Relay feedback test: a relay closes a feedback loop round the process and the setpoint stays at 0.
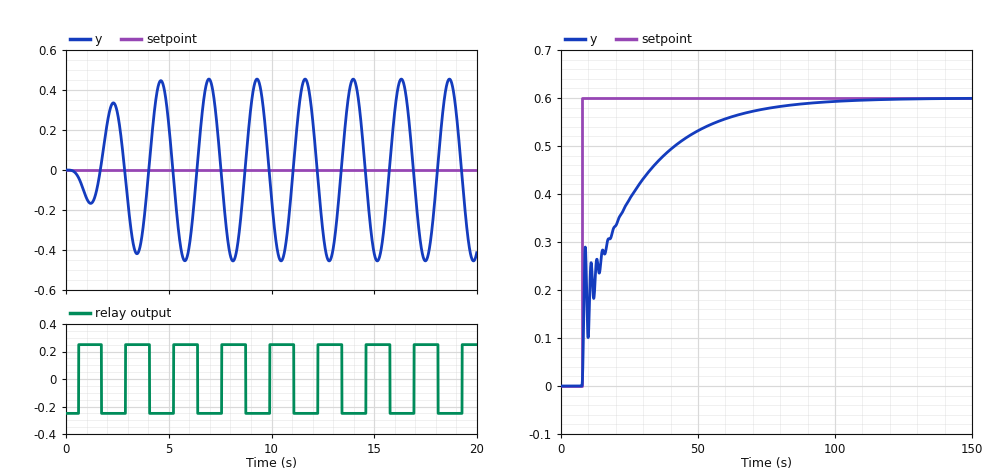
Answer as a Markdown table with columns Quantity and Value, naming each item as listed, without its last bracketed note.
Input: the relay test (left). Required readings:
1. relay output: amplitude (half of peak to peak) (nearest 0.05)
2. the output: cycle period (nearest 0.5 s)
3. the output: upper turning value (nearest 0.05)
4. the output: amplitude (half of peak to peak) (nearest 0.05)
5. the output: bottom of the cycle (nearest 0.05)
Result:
| Quantity | Value |
|---|---|
| relay output: amplitude (half of peak to peak) | 0.25 |
| the output: cycle period | 2.5 s |
| the output: upper turning value | 0.45 |
| the output: amplitude (half of peak to peak) | 0.45 |
| the output: bottom of the cycle | -0.45 |
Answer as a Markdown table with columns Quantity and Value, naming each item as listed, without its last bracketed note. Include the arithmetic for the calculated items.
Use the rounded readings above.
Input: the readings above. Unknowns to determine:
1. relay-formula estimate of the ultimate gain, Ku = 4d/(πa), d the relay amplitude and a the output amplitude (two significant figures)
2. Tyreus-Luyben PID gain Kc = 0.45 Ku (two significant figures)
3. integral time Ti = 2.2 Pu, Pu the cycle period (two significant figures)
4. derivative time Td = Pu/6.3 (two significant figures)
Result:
| Quantity | Value |
|---|---|
| relay-formula estimate of the ultimate gain, Ku = 4d/(πa), d the relay amplitude and a the output amplitude | 4 × 0.25 / (π × 0.45) = 0.71 |
| Tyreus-Luyben PID gain Kc = 0.45 Ku | 0.45 × 0.71 = 0.32 |
| integral time Ti = 2.2 Pu, Pu the cycle period | 2.2 × 2.5 = 5.5 s |
| derivative time Td = Pu/6.3 | 2.5 / 6.3 = 0.40 s |
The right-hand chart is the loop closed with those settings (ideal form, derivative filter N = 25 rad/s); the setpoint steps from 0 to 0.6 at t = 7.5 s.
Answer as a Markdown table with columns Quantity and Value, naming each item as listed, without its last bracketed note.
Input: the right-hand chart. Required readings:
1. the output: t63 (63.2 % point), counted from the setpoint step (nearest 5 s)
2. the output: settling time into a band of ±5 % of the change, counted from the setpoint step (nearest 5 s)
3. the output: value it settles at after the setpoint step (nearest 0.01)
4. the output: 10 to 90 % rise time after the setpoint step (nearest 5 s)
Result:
| Quantity | Value |
|---|---|
| the output: t63 (63.2 % point), counted from the setpoint step | 15 s |
| the output: settling time into a band of ±5 % of the change, counted from the setpoint step | 60 s |
| the output: value it settles at after the setpoint step | 0.60 |
| the output: 10 to 90 % rise time after the setpoint step | 45 s |
